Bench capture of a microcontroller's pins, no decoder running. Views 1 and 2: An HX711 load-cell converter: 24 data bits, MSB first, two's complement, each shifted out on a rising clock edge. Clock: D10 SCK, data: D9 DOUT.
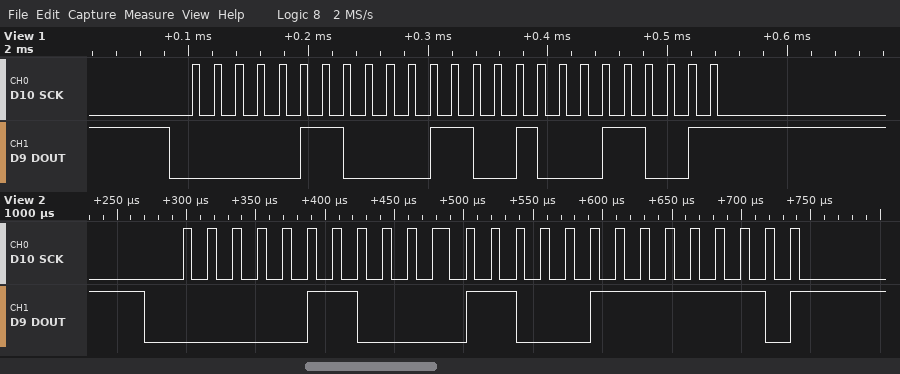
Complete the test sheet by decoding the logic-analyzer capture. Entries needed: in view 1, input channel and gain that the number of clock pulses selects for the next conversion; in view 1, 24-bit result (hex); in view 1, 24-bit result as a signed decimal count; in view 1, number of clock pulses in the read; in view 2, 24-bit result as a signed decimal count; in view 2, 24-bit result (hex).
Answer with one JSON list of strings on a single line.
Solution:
["channel A, gain 128", "0x061919", "399641", "25", "399614", "0x0618FE"]
